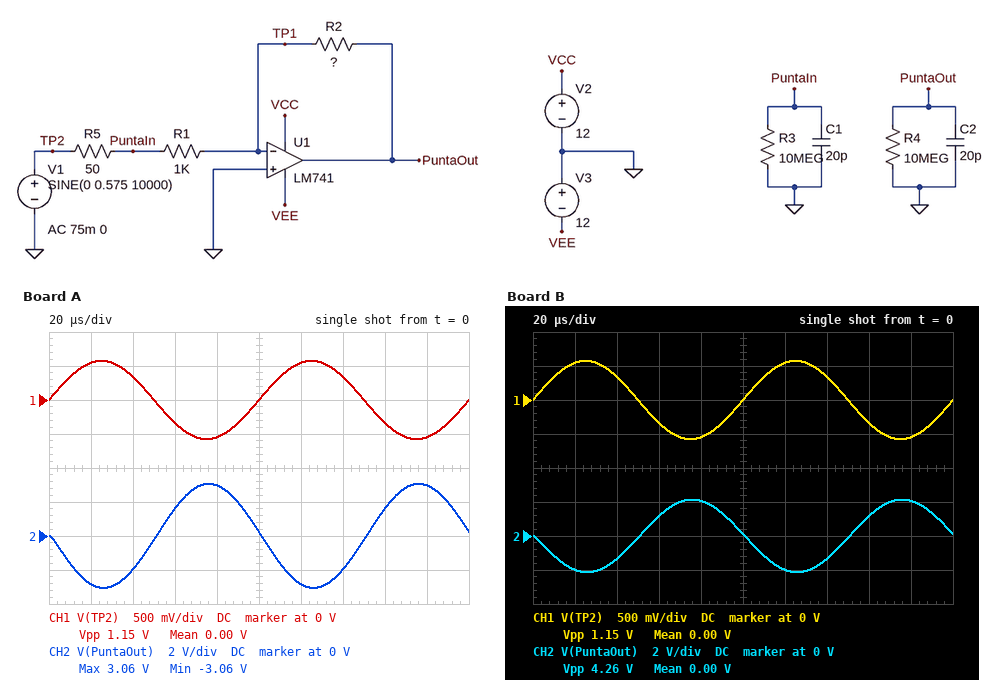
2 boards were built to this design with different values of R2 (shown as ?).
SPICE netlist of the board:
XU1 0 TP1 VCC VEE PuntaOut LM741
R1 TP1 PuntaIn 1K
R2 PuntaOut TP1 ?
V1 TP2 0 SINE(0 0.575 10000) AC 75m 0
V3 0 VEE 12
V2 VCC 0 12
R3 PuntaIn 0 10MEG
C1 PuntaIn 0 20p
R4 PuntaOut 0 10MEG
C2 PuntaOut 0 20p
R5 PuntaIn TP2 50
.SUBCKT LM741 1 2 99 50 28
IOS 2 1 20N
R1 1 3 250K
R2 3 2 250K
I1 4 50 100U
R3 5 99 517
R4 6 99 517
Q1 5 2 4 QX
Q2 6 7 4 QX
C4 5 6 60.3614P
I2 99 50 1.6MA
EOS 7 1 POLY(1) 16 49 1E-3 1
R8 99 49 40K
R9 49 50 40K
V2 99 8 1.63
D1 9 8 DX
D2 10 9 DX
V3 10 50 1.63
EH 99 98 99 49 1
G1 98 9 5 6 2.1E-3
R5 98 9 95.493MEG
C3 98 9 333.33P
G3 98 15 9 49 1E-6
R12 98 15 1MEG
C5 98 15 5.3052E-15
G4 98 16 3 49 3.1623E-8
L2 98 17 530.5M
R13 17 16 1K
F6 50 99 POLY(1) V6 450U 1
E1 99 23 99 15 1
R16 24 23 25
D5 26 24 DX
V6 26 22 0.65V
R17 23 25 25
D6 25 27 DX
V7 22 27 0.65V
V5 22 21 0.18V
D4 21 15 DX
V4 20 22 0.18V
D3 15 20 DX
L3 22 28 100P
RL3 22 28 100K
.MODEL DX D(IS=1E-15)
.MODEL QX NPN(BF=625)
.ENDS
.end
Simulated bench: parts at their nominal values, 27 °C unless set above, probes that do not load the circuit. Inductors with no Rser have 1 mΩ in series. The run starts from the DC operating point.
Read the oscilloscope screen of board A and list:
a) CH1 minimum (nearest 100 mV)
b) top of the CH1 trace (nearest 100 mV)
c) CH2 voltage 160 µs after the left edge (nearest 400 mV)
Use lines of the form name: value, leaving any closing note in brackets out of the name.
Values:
CH1 minimum: -600 mV
top of the CH1 trace: 600 mV
CH2 voltage 160 µs after the left edge: 1.6 V
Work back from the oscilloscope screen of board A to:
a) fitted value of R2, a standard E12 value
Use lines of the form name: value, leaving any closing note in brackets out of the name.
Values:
fitted value of R2, a standard E12 value: 5.6 kΩ
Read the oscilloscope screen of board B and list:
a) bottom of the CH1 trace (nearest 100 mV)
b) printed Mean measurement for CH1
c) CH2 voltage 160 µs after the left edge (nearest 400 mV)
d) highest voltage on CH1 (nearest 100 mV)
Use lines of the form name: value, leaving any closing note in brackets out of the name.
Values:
bottom of the CH1 trace: -600 mV
printed Mean measurement for CH1: 0.00 V
CH2 voltage 160 µs after the left edge: 1.2 V
highest voltage on CH1: 600 mV
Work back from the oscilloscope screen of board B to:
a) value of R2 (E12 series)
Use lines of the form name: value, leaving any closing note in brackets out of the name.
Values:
value of R2: 3.9 kΩ
